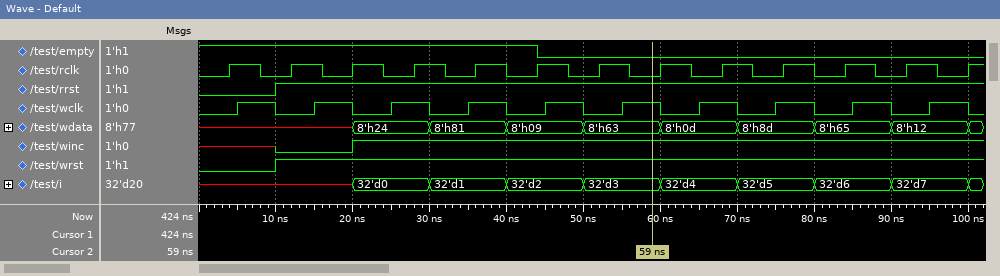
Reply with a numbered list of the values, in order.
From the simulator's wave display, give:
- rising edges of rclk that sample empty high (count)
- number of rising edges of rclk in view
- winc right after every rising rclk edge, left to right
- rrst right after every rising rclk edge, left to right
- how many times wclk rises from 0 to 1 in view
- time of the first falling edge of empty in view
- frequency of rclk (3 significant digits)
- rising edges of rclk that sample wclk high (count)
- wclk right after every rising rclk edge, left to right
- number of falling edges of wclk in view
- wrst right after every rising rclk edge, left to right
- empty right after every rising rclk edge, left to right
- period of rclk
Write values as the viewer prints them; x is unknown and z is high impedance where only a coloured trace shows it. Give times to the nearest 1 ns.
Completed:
1. 6
2. 13
3. x 0 1 1 1 1 1 1 1 1 1 1 1
4. 0 1 1 1 1 1 1 1 1 1 1 1 1
5. 10
6. 44 ns
7. 125 MHz
8. 7
9. 0 0 0 1 1 0 0 0 1 1 0 0 0
10. 10
11. 0 1 1 1 1 1 1 1 1 1 1 1 1
12. 1 1 1 1 1 0 0 0 0 0 0 0 0
13. 8 ns
